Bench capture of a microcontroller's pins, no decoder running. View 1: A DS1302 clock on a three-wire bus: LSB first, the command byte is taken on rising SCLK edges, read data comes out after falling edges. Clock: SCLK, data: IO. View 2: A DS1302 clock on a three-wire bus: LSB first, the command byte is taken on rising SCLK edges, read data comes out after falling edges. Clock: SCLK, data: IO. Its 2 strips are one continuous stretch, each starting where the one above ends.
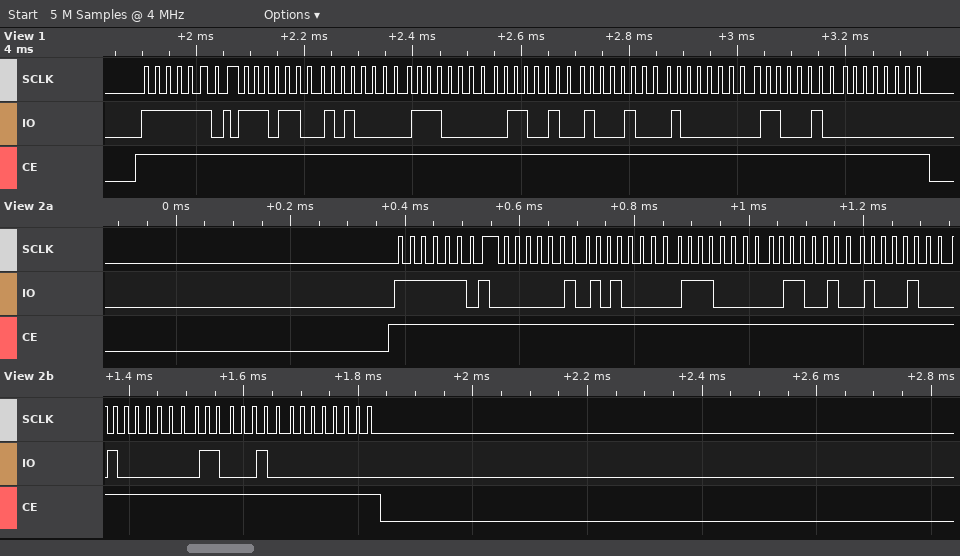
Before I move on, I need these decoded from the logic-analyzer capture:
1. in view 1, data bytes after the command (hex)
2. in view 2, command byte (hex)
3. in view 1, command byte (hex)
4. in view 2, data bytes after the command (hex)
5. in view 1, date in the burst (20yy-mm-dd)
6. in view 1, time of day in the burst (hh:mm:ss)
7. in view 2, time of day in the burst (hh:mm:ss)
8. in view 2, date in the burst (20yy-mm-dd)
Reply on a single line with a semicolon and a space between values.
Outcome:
37 05 07 26 11 01 23 00; 0xBF; 0xBF; 40 05 07 26 11 01 23 00; 2023-11-26; 07:05:37; 07:05:40; 2023-11-26
